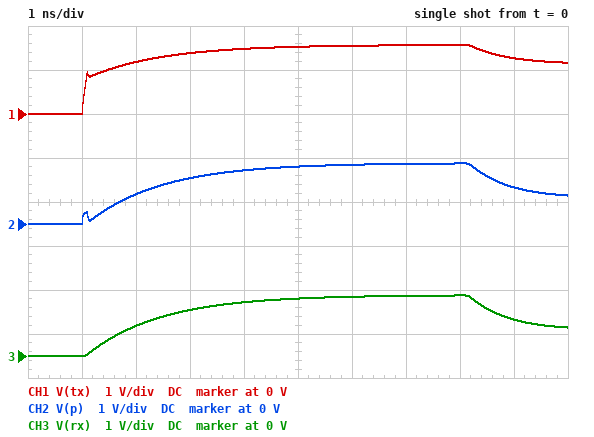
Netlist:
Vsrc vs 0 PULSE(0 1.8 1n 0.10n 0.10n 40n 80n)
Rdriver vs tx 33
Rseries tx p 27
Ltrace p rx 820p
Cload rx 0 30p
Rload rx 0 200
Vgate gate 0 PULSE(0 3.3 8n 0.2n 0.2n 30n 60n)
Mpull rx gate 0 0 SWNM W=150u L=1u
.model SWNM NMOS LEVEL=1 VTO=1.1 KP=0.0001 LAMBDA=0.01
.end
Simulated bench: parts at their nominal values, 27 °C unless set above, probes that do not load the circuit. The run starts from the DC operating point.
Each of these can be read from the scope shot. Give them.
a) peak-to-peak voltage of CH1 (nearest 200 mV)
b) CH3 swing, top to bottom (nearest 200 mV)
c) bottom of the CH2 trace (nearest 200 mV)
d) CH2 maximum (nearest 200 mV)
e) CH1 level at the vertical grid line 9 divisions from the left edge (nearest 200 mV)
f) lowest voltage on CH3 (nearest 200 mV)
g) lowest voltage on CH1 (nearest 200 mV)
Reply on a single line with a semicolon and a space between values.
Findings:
1.6 V; 1.4 V; 0 V; 1.4 V; 1.2 V; 0 V; 0 V
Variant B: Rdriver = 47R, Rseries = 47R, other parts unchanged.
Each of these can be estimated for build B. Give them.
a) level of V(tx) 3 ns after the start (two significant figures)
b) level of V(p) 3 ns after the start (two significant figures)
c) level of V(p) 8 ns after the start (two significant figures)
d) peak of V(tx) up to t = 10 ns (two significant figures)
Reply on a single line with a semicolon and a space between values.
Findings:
1.3 V; 780 mV; 1.2 V; 1.5 V
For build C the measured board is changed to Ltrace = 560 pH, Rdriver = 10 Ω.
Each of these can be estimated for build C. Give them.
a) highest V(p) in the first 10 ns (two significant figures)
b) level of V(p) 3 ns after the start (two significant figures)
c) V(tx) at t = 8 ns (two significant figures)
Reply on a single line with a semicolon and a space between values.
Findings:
1.5 V; 1.3 V; 1.7 V
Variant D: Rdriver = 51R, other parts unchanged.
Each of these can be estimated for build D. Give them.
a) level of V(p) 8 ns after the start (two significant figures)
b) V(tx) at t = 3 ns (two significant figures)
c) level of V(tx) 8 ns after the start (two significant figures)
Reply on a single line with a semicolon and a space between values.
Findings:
1.3 V; 1.2 V; 1.5 V
